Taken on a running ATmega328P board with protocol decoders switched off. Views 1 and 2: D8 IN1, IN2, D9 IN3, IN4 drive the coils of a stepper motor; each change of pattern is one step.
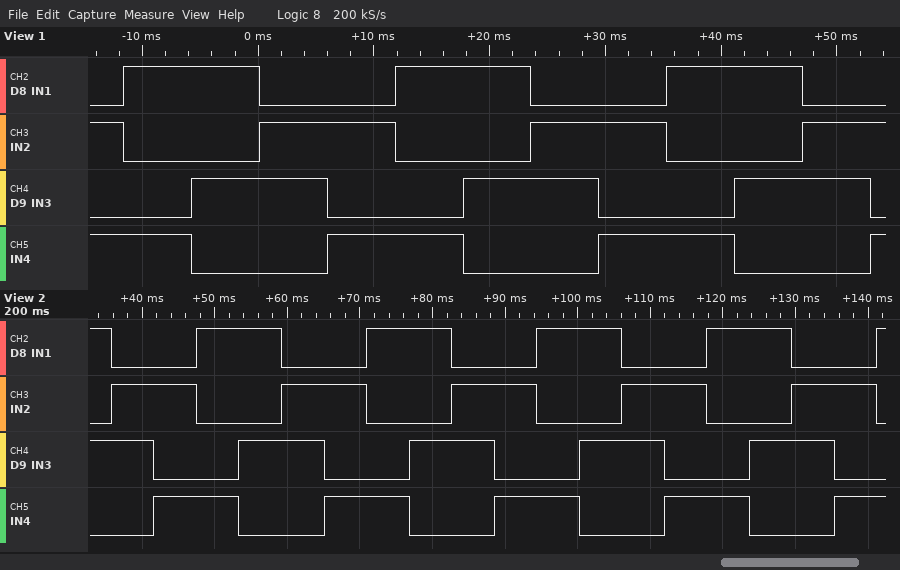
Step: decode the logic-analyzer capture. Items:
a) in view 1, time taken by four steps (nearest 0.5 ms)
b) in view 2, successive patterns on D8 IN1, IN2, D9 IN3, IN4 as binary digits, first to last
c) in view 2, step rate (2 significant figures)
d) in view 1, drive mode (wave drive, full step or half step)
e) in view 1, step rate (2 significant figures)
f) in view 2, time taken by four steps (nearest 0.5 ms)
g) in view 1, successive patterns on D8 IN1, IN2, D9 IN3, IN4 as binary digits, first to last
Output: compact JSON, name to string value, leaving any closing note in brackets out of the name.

{"in view 1, time taken by four steps": "23.5 ms", "in view 2, successive patterns on D8 IN1, IN2, D9 IN3, IN4 as binary digits, first to last": "1010 0110 0101 1001 1010 0110 0101 1001 1010 0110 0101 1001 1010 0110 0101 1001 1010 0110 0101 1001", "in view 2, step rate": "170 steps/s", "in view 1, drive mode": "full step", "in view 1, step rate": "170 steps/s", "in view 2, time taken by four steps": "23.5 ms", "in view 1, successive patterns on D8 IN1, IN2, D9 IN3, IN4 as binary digits, first to last": "0101 1001 1010 0110 0101 1001 1010 0110 0101 1001 1010 0110 0101"}
